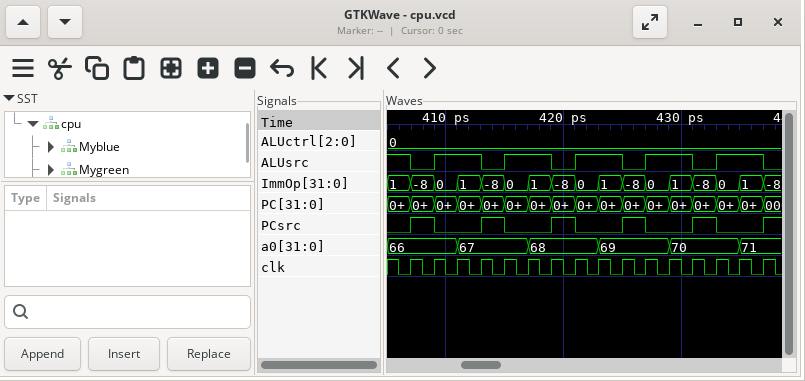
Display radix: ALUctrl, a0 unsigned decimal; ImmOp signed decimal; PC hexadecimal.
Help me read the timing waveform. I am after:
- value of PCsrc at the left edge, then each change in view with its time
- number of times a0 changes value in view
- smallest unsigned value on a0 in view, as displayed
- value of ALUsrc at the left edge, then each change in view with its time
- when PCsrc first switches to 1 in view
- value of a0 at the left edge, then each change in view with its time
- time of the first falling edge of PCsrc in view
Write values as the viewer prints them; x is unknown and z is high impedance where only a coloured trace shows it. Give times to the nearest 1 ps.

0, 1 at 407 ps, 0 at 409 ps, 1 at 413 ps, 0 at 415 ps, 1 at 419 ps, 0 at 421 ps, 1 at 425 ps, 0 at 427 ps, 1 at 431 ps, 0 at 433 ps, 1 at 437 ps
5
66
1, 0 at 407 ps, 1 at 409 ps, 0 at 413 ps, 1 at 415 ps, 0 at 419 ps, 1 at 421 ps, 0 at 425 ps, 1 at 427 ps, 0 at 431 ps, 1 at 433 ps, 0 at 437 ps
407 ps
66, 67 at 411 ps, 68 at 417 ps, 69 at 423 ps, 70 at 429 ps, 71 at 435 ps
409 ps
